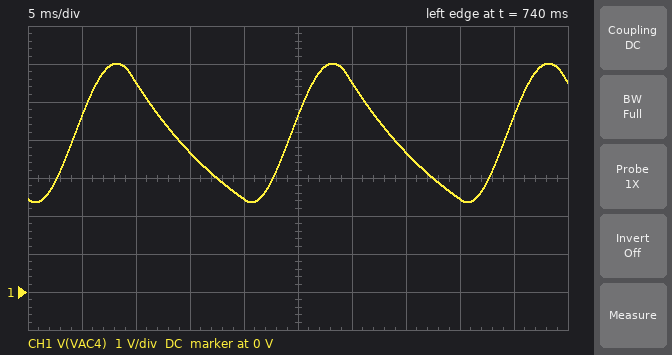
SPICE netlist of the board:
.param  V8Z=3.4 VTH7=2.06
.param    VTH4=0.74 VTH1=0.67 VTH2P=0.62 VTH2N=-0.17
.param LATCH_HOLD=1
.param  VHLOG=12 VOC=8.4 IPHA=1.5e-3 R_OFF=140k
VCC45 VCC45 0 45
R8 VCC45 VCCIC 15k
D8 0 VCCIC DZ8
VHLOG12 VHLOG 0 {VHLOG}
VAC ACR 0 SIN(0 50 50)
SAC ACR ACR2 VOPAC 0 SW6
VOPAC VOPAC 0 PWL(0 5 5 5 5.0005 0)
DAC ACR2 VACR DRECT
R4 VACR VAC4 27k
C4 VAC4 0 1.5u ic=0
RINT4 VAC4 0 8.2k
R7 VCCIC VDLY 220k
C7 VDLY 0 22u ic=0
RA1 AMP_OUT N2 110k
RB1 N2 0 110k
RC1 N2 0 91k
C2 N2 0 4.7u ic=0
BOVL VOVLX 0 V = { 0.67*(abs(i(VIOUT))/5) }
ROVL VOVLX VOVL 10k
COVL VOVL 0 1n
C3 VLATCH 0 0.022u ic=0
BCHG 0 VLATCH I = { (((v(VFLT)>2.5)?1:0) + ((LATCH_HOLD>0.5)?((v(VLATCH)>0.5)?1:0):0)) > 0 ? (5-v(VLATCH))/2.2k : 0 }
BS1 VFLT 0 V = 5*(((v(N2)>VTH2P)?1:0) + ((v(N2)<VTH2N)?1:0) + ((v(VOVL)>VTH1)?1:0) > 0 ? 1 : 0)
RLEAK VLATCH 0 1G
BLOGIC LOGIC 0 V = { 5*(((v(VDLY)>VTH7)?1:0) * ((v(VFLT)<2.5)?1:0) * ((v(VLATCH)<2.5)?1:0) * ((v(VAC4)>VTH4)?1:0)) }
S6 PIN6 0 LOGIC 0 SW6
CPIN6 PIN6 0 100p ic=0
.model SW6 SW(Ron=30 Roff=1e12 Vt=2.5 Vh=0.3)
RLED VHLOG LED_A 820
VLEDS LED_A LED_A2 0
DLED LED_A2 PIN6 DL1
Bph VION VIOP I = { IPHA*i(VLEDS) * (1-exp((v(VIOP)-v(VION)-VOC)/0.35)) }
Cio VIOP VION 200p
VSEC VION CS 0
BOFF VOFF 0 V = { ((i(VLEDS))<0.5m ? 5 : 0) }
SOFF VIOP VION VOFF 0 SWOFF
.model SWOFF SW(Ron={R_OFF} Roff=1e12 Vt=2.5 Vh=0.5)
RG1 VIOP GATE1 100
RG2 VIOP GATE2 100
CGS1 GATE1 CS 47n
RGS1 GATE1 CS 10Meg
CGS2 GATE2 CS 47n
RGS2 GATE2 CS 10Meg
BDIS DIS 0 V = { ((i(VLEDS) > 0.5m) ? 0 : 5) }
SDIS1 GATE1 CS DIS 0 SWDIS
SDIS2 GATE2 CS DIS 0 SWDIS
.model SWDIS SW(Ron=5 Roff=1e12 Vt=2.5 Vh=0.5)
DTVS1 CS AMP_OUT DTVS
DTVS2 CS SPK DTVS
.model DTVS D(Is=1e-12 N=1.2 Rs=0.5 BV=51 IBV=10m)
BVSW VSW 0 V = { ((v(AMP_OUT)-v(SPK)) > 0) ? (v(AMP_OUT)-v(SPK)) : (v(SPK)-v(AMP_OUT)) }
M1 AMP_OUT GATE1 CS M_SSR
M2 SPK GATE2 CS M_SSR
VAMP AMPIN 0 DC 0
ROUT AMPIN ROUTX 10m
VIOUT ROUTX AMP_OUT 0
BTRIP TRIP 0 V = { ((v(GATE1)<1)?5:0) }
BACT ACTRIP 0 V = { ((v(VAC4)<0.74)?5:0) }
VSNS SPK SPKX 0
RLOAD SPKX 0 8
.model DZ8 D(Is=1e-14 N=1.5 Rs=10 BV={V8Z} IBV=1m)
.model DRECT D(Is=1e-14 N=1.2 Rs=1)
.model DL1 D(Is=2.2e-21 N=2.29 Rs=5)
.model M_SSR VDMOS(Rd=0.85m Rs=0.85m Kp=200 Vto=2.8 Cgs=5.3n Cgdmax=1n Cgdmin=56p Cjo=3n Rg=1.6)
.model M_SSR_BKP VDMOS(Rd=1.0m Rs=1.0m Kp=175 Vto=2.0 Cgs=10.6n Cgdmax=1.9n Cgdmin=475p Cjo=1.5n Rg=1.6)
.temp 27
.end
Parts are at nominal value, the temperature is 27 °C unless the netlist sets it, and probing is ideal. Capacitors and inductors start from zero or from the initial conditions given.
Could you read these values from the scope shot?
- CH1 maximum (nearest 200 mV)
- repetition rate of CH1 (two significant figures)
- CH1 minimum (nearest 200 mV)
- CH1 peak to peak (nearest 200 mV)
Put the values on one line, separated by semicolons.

6.0 V; 50 Hz; 2.4 V; 3.6 V
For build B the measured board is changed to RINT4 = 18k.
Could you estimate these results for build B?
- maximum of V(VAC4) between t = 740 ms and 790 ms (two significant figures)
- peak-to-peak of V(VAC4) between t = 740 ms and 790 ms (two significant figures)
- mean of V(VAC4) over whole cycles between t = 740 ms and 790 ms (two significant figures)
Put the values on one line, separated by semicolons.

9.6 V; 3.4 V; 7.8 V
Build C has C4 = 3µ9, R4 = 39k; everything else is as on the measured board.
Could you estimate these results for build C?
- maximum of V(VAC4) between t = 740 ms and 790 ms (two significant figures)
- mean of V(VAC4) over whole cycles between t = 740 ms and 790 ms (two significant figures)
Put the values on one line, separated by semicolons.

3.5 V; 3.0 V
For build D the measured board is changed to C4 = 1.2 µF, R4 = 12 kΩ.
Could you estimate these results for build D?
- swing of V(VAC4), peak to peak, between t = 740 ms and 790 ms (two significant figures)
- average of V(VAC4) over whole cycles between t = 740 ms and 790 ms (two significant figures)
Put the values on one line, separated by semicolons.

8.8 V; 7.8 V
